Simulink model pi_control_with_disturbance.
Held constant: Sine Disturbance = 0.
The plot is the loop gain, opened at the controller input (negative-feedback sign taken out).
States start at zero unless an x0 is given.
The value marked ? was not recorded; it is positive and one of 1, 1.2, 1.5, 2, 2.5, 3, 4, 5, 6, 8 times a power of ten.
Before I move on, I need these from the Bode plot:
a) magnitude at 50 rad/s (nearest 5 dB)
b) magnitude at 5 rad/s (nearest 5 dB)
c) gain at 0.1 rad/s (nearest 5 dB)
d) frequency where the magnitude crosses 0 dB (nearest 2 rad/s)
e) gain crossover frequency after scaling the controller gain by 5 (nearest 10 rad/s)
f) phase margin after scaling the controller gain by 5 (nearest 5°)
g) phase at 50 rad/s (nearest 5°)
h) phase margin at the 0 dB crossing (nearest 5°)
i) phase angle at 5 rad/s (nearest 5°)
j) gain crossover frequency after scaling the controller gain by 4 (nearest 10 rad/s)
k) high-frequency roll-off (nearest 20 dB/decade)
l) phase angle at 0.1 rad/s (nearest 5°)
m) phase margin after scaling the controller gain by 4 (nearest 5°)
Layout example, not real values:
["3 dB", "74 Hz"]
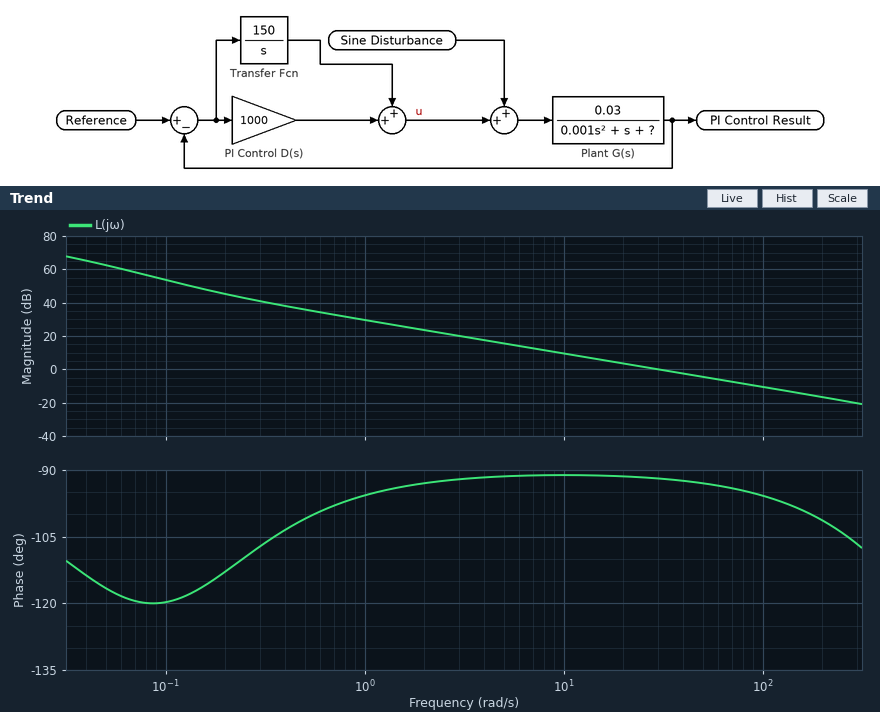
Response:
["-5 dB", "15 dB", "55 dB", "30 rad/s", "150 rad/s", "80°", "-95°", "90°", "-90°", "120 rad/s", "-20 dB/decade", "-120°", "85°"]
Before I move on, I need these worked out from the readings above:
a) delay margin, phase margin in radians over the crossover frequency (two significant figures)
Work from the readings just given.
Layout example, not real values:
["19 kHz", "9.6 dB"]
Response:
["0.052 s"]
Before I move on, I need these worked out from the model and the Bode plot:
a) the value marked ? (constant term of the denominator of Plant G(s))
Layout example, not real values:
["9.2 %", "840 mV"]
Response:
["0.05"]
